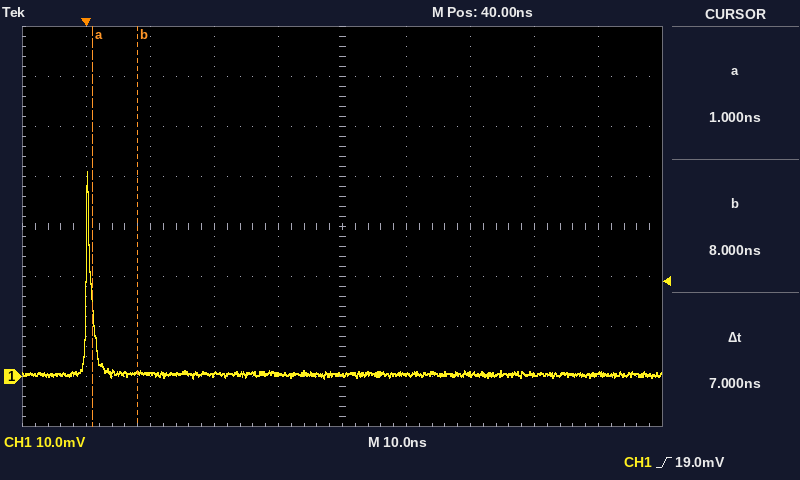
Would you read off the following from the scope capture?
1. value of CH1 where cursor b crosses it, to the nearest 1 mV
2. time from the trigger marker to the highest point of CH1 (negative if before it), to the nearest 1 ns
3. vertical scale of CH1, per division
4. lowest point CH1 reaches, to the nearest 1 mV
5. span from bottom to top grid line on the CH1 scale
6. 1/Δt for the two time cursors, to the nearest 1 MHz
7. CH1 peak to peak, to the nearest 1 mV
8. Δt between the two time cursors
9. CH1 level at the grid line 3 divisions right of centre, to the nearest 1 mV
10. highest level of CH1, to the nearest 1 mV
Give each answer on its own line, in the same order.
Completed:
1 mV
0 ns
10 mV
0 mV
80 mV
143 MHz
41 mV
7 ns
0 mV
41 mV
